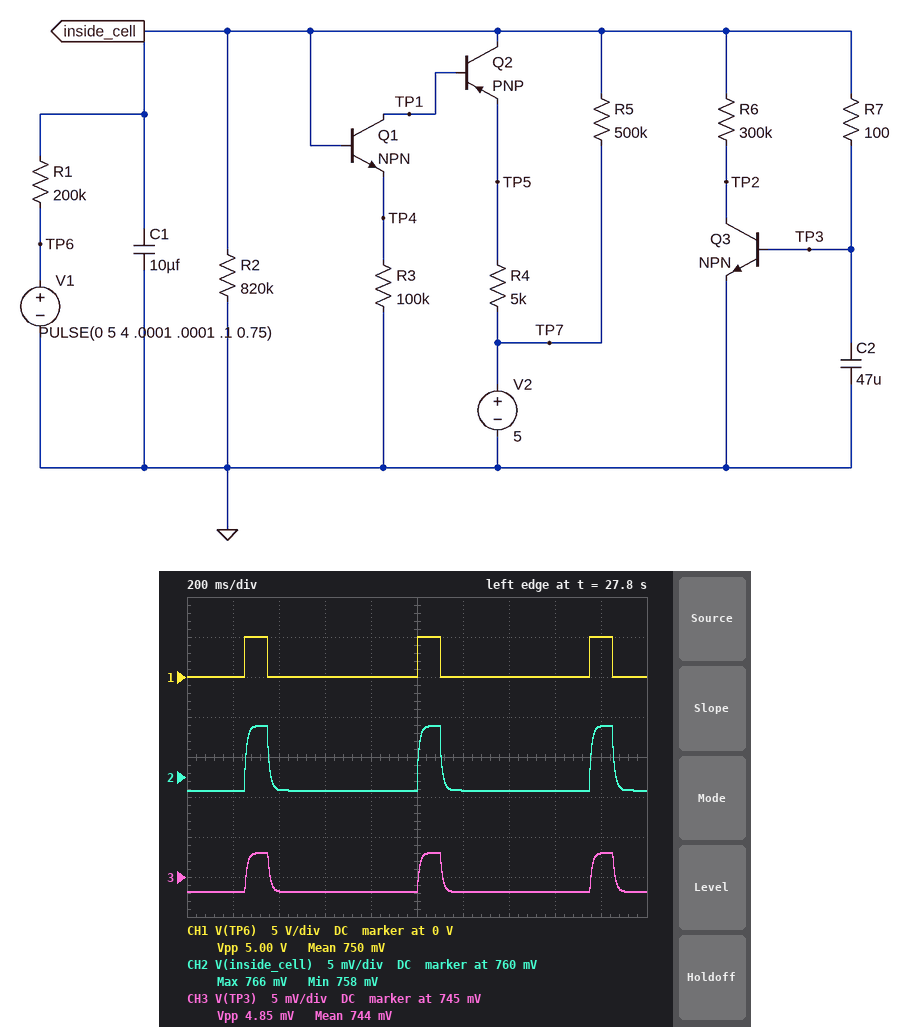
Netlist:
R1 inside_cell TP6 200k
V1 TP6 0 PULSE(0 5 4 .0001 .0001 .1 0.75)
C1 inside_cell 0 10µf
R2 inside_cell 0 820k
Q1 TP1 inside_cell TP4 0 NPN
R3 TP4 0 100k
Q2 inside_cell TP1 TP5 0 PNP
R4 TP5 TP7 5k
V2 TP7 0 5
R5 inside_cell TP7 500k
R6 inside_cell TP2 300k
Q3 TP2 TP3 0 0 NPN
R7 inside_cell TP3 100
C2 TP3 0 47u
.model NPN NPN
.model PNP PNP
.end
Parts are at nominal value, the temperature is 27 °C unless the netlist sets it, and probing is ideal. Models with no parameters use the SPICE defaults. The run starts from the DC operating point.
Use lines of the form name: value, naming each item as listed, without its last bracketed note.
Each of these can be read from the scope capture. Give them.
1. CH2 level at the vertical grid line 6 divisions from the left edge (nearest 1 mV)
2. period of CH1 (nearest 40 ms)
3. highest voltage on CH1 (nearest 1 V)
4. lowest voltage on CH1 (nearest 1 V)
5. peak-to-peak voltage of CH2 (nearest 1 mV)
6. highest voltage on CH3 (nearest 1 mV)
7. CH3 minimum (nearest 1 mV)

CH2 level at the vertical grid line 6 divisions from the left edge: 758 mV
period of CH1: 760 ms
highest voltage on CH1: 5 V
lowest voltage on CH1: 0 V
peak-to-peak voltage of CH2: 8 mV
highest voltage on CH3: 748 mV
CH3 minimum: 743 mV
